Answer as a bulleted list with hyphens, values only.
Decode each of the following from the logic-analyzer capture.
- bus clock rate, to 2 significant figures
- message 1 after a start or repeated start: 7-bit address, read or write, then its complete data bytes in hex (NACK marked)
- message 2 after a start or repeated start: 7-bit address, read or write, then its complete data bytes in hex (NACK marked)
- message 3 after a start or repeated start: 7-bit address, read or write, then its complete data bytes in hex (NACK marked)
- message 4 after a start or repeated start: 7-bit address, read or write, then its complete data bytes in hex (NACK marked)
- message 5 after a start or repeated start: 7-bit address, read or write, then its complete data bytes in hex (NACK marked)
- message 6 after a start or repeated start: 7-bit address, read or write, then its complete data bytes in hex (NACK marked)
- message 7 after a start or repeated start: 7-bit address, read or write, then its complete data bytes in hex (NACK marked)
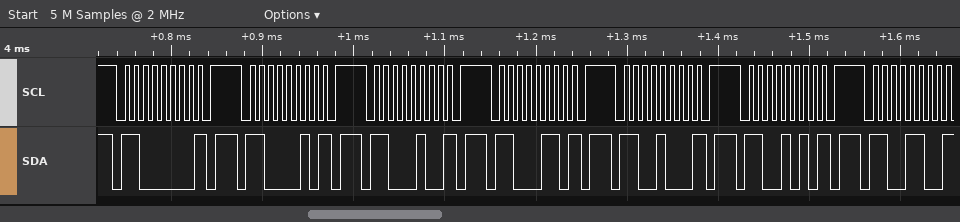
- 100 kHz
- 0x60 write NACK
- 0x61 write NACK
- 0x62 write NACK
- 0x63 write NACK
- 0x64 write NACK
- 0x65 write NACK
- 0x66 write NACK
